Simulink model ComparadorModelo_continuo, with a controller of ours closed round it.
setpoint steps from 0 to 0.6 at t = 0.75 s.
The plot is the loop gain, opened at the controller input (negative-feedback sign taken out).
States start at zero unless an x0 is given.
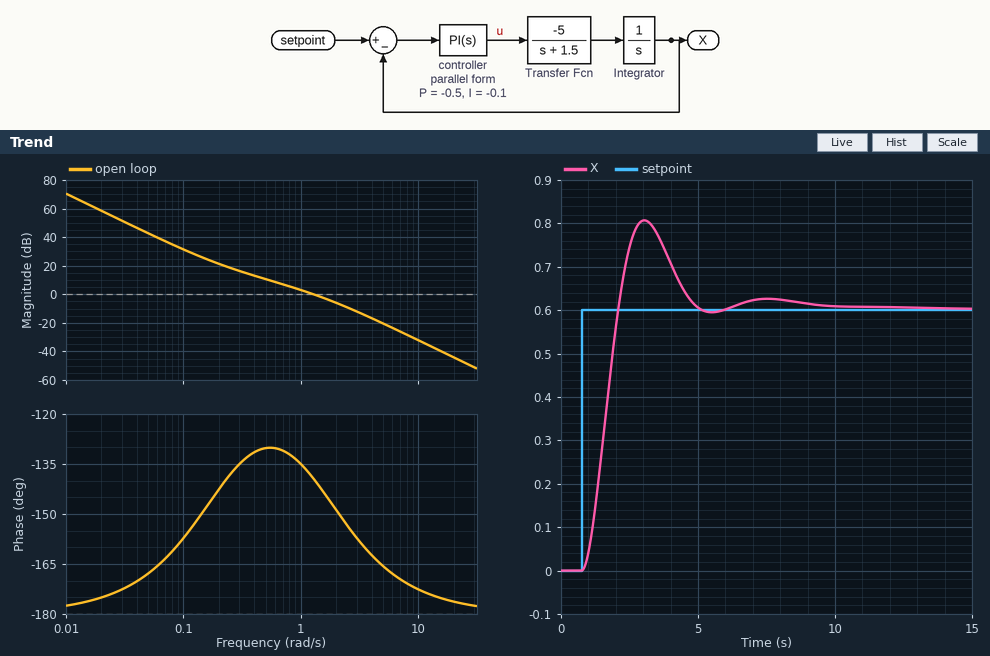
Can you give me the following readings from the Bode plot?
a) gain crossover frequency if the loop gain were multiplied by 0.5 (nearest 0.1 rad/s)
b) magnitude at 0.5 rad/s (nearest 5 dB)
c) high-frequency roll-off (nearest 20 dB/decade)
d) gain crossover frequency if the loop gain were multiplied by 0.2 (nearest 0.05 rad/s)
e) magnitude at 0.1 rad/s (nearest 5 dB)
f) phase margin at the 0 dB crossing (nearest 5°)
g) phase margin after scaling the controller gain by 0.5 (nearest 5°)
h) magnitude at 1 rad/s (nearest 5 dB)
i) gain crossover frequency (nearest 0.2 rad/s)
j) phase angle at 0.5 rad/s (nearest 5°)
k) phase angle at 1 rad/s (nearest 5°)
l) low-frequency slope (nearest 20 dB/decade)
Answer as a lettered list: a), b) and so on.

a) 0.8 rad/s
b) 10 dB
c) -40 dB/decade
d) 0.35 rad/s
e) 30 dB
f) 40°
g) 50°
h) 5 dB
i) 1.2 rad/s
j) -130°
k) -135°
l) -40 dB/decade
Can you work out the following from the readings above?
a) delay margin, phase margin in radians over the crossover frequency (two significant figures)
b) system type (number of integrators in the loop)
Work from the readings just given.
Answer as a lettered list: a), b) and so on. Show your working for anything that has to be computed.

a) 40 × π / 180 / 1.2 = 0.58 s
b) 2
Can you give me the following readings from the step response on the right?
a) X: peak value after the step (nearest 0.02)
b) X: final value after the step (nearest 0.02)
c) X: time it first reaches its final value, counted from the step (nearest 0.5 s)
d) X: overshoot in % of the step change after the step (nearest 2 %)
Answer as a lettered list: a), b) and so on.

a) 0.80
b) 0.60
c) 1.5 s
d) 34 %
